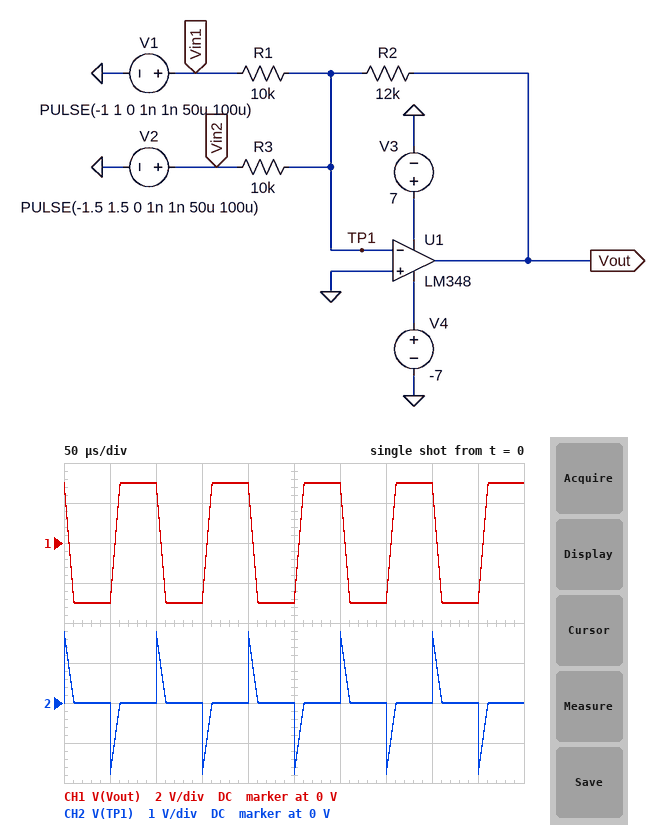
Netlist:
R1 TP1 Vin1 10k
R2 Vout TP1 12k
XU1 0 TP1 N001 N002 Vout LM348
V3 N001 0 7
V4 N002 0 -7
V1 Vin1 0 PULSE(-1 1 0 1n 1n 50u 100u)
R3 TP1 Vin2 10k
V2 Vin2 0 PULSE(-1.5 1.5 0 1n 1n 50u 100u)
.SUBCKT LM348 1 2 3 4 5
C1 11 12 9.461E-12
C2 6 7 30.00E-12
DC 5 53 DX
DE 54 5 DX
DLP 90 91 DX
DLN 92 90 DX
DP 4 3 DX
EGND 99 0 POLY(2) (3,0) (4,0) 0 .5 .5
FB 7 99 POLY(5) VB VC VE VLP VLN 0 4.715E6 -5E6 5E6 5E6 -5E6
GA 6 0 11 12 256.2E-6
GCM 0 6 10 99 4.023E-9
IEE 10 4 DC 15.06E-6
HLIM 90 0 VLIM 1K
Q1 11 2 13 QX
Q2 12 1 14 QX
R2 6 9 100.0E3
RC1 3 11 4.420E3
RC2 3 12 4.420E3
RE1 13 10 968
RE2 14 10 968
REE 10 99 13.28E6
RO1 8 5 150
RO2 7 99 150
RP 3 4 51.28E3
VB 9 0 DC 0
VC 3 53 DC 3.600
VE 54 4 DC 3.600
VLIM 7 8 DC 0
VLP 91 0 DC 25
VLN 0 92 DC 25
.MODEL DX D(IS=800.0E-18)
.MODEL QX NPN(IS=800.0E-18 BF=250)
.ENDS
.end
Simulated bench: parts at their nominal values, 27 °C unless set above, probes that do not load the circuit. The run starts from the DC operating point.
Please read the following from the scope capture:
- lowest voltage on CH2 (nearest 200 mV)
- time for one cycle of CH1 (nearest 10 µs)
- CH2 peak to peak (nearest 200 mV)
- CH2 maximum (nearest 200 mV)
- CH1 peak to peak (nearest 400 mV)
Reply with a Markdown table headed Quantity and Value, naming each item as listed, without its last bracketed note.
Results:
| Quantity | Value |
|---|---|
| lowest voltage on CH2 | -1.8 V |
| time for one cycle of CH1 | 100 µs |
| CH2 peak to peak | 3.6 V |
| CH2 maximum | 1.8 V |
| CH1 peak to peak | 6.0 V |
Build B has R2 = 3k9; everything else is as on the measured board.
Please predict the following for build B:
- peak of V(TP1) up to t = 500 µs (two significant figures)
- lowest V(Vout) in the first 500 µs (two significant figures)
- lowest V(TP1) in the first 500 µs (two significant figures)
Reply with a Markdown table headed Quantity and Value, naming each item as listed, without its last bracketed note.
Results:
| Quantity | Value |
|---|---|
| peak of V(TP1) up to t = 500 µs | 1.1 V |
| lowest V(Vout) in the first 500 µs | -1.0 V |
| lowest V(TP1) in the first 500 µs | -1.1 V |
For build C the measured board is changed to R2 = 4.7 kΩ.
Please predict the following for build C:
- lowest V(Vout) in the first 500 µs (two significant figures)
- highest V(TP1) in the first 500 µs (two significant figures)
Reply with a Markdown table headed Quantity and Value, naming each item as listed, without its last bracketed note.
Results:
| Quantity | Value |
|---|---|
| lowest V(Vout) in the first 500 µs | -1.2 V |
| highest V(TP1) in the first 500 µs | 1.2 V |
